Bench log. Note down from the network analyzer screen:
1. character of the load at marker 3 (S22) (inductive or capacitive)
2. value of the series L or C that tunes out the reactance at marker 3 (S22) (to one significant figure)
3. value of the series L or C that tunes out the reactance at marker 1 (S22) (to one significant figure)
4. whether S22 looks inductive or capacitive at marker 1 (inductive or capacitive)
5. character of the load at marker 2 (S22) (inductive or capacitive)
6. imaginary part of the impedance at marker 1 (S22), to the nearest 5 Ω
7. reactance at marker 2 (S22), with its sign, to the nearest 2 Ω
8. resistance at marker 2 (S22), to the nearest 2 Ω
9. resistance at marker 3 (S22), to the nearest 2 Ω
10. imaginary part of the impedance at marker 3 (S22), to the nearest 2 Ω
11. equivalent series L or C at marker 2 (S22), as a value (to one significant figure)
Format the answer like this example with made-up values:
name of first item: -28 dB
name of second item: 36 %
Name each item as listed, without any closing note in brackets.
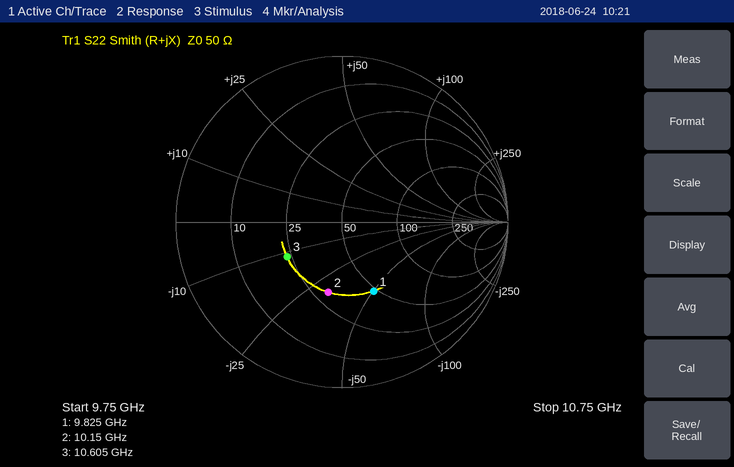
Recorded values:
character of the load at marker 3 (S22): capacitive
value of the series L or C that tunes out the reactance at marker 3 (S22): 200 pH
value of the series L or C that tunes out the reactance at marker 1 (S22): 800 pH
whether S22 looks inductive or capacitive at marker 1: capacitive
character of the load at marker 2 (S22): capacitive
imaginary part of the impedance at marker 1 (S22), to the nearest 5 Ω: -50 Ω
reactance at marker 2 (S22), with its sign, to the nearest 2 Ω: -32 Ω
resistance at marker 2 (S22), to the nearest 2 Ω: 30 Ω
resistance at marker 3 (S22), to the nearest 2 Ω: 24 Ω
imaginary part of the impedance at marker 3 (S22), to the nearest 2 Ω: -12 Ω
equivalent series L or C at marker 2 (S22), as a value: 500 fF
